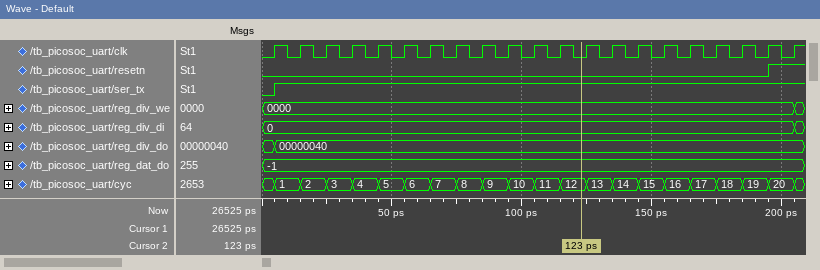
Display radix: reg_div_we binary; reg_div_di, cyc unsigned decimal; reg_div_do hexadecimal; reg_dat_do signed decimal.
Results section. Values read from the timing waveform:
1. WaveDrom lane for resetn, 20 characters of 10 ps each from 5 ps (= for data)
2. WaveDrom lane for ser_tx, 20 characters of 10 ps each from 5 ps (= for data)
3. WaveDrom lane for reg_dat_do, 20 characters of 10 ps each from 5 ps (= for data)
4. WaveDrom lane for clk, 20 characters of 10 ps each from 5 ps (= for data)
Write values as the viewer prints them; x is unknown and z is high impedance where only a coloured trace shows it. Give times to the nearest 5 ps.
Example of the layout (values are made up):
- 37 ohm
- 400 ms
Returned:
- {name: 'resetn', wave: '0..................1'}
- {name: 'ser_tx', wave: '1...................'}
- {name: 'reg_dat_do', wave: '=...................', data: '-1'}
- {name: 'clk', wave: 'p...................'}
